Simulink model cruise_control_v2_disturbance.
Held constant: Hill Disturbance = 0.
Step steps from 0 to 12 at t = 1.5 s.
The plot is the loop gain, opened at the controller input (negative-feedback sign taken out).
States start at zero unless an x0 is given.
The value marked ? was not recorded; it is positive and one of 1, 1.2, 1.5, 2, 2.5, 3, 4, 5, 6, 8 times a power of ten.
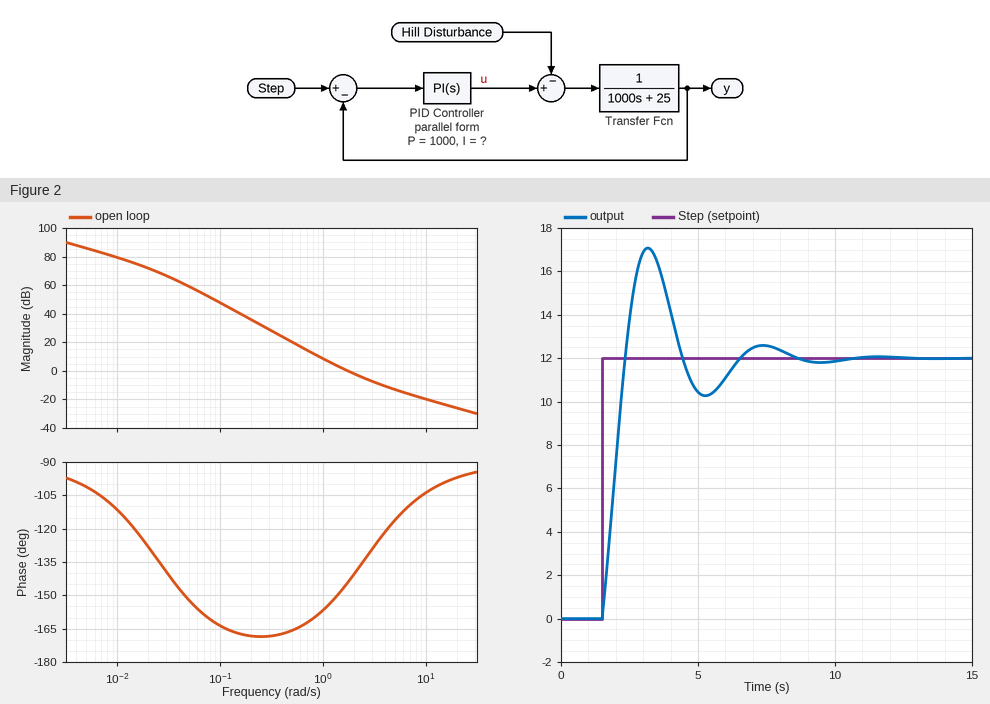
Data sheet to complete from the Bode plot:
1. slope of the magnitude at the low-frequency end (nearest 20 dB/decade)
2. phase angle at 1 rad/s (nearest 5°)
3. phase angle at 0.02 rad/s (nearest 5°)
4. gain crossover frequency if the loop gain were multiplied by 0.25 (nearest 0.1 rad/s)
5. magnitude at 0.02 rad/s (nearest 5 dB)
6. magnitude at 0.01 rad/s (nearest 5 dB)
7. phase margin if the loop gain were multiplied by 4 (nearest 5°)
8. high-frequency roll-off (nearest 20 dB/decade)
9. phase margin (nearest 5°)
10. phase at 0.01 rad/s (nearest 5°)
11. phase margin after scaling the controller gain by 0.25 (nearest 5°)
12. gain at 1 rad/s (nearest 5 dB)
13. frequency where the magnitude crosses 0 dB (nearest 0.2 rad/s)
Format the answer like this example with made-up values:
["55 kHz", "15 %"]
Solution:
["-20 dB/decade", "-155°", "-130°", "0.8 rad/s", "70 dB", "80 dB", "60°", "-20 dB/decade", "35°", "-110°", "20°", "10 dB", "1.8 rad/s"]
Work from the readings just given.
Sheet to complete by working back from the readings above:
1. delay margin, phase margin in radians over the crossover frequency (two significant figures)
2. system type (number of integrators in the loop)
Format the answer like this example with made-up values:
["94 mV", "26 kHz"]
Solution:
["0.34 s", "1"]
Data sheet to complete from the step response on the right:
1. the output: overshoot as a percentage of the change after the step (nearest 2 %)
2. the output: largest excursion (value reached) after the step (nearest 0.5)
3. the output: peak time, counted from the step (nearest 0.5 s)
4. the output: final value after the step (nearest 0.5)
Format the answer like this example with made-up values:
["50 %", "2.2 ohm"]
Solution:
["42 %", "17.0", "1.5 s", "12.0"]
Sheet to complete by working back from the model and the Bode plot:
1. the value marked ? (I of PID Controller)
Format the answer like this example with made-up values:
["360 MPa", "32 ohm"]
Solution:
["2500"]
